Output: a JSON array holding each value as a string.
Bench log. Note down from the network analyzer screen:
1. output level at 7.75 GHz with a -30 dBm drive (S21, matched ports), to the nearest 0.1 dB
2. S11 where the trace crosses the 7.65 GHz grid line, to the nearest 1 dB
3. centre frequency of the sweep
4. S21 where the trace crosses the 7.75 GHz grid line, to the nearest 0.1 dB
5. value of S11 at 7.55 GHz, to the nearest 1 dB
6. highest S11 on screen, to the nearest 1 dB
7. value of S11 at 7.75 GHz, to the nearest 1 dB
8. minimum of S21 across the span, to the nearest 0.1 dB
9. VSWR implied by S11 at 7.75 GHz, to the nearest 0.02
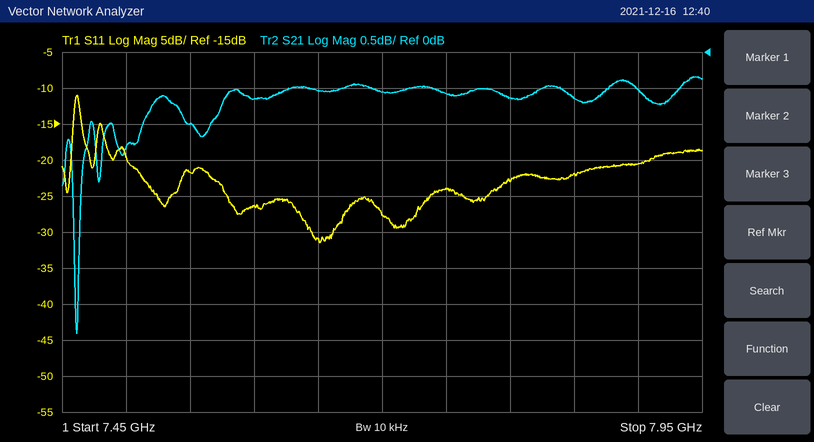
["-30.6 dBm", "-31 dB", "7.7 GHz", "-0.6 dB", "-22 dB", "-11 dB", "-24 dB", "-3.9 dB", "1.14"]
